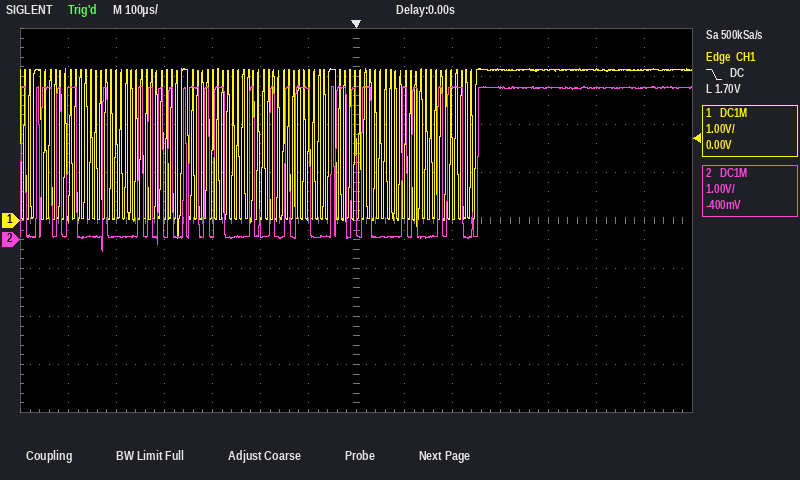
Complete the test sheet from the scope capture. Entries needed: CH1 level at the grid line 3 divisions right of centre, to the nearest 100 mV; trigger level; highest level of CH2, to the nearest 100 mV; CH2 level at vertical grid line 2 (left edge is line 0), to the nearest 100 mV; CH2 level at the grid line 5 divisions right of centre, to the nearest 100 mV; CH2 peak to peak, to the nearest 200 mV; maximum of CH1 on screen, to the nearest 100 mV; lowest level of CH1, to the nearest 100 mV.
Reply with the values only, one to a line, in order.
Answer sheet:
3.1 V
1.70 V
3.2 V
100 mV
3.2 V
3.4 V
3.2 V
-400 mV
